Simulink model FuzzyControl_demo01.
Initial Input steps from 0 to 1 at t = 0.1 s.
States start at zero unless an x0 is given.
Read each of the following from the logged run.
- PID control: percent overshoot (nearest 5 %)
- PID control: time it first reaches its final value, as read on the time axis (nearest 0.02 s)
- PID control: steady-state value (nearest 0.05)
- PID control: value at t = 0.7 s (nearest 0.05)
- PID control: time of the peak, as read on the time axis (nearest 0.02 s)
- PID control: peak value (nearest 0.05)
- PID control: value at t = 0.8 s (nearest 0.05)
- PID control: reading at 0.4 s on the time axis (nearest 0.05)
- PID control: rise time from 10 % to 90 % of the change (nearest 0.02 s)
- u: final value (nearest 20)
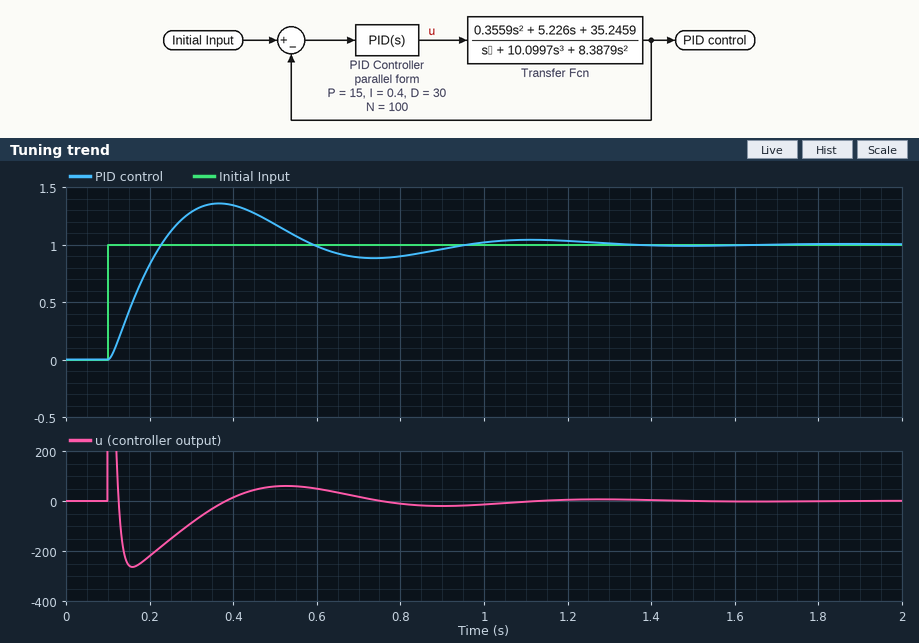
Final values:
35 %
0.22 s
1.00
0.90
0.36 s
1.35
0.90
1.35
0.10 s
0
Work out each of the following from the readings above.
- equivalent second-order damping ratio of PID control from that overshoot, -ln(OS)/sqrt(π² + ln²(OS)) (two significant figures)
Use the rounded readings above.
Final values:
0.32
